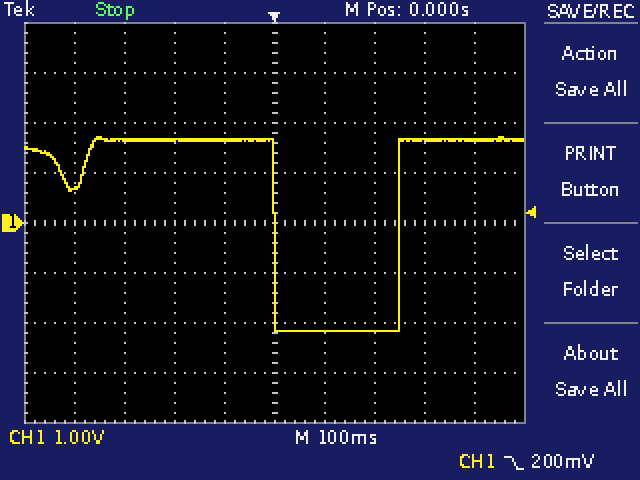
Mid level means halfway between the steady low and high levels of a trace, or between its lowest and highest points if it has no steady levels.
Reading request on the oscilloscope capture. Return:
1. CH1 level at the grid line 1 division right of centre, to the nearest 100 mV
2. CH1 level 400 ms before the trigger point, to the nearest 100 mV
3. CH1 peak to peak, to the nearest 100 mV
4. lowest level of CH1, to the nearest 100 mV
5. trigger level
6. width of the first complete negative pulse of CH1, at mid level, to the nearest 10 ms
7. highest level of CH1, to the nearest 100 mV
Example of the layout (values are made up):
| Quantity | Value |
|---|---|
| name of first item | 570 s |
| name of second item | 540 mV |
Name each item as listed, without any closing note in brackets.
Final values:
| Quantity | Value |
|---|---|
| CH1 level at the grid line 1 division right of centre, to the nearest 100 mV | -2.2 V |
| CH1 level 400 ms before the trigger point, to the nearest 100 mV | 700 mV |
| CH1 peak to peak, to the nearest 100 mV | 3.9 V |
| lowest level of CH1, to the nearest 100 mV | -2.2 V |
| trigger level | 200 mV |
| width of the first complete negative pulse of CH1, at mid level, to the nearest 10 ms | 250 ms |
| highest level of CH1, to the nearest 100 mV | 1.7 V |
